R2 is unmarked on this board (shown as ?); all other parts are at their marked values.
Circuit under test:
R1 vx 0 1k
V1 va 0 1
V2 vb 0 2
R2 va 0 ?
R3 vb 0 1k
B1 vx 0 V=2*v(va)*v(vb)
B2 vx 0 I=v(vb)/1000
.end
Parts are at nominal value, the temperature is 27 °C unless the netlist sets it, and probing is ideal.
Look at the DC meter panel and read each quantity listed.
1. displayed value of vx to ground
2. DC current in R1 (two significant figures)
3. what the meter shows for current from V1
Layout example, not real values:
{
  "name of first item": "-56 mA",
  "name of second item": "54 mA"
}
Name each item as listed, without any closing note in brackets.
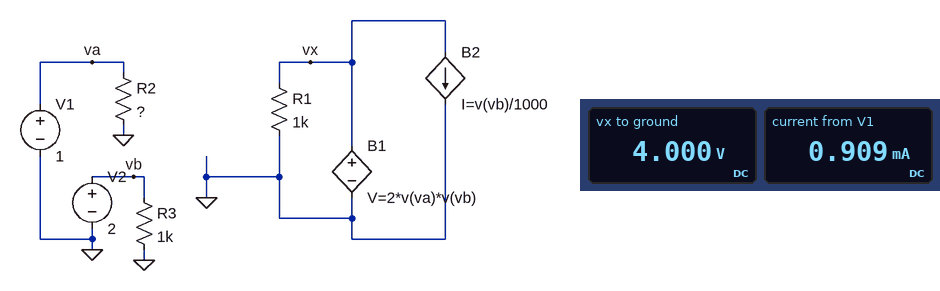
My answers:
{
  "displayed value of vx to ground": "4.000 V",
  "DC current in R1": "4.0 mA",
  "what the meter shows for current from V1": "0.909 mA"
}
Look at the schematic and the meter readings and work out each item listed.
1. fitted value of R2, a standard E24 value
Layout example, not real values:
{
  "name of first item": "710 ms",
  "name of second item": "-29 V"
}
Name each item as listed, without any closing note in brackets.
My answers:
{
  "fitted value of R2, a standard E24 value": "1.1 kΩ"
}
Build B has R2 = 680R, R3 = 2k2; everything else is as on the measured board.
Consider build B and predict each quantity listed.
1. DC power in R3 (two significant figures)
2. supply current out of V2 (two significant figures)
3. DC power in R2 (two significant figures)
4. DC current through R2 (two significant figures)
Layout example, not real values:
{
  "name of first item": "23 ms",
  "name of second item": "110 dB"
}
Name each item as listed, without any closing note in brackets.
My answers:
{
  "DC power in R3": "1.8 mW",
  "supply current out of V2": "910 µA",
  "DC power in R2": "1.5 mW",
  "DC current through R2": "1.5 mA"
}
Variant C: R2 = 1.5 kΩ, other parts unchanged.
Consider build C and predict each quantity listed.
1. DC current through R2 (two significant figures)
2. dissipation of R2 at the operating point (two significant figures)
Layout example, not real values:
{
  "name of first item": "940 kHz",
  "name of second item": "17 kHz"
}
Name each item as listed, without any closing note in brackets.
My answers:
{
  "DC current through R2": "670 µA",
  "dissipation of R2 at the operating point": "670 µW"
}
